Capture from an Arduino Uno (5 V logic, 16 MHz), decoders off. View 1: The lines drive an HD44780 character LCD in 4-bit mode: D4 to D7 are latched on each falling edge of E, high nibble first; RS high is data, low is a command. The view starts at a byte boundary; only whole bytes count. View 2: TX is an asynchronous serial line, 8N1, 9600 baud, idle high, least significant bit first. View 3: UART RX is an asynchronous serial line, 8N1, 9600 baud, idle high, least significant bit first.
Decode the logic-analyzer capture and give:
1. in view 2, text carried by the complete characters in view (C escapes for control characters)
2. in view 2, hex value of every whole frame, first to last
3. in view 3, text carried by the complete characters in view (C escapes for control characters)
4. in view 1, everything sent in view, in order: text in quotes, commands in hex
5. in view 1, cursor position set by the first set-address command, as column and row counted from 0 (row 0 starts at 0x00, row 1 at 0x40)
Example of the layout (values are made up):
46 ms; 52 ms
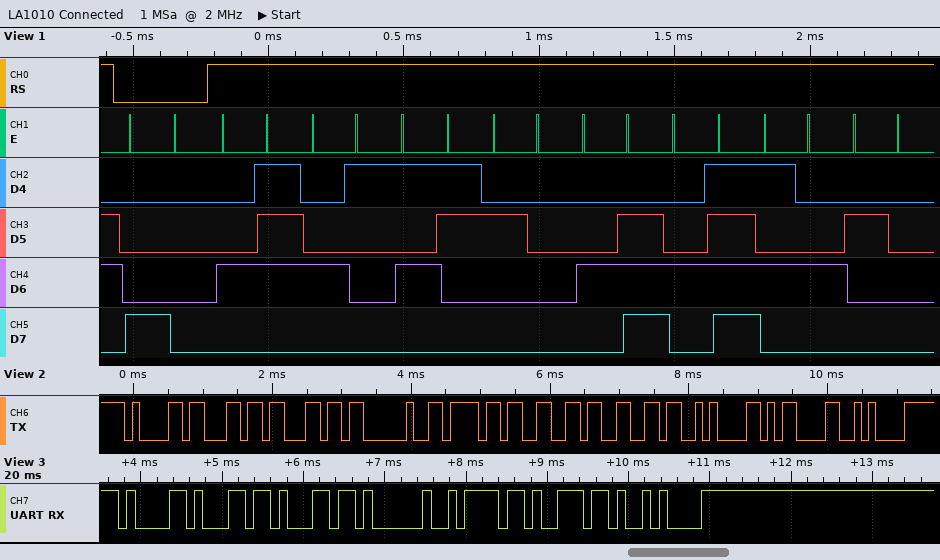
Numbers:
"all off\n\r\n"; 61 6C 6C 20 6F 66 66 0A 0D 0A; "all on\n"; 0x80 "GAS NOT "; column 0, row 0
